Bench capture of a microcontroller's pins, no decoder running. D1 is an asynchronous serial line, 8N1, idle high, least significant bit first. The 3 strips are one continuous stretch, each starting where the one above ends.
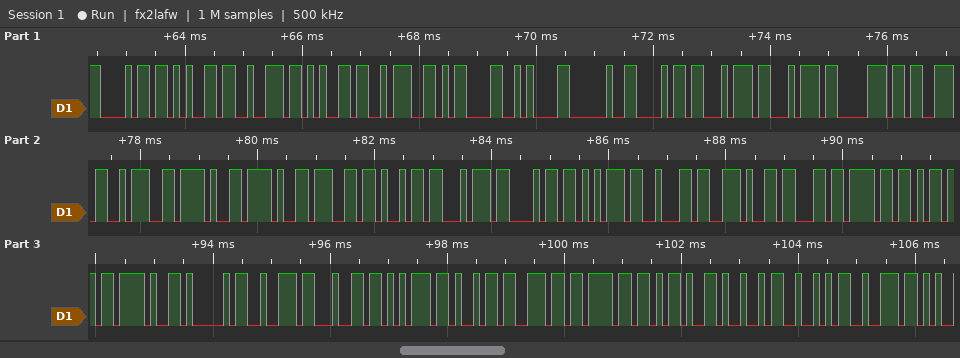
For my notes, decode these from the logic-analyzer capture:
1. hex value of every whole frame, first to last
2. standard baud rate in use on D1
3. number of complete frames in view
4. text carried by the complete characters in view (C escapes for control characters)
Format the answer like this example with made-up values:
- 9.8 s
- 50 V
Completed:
- 0x68 0x65 0x72 0x65 0x3A 0x0D 0x0A 0x20 0x68 0x74 0x74 0x70 0x73 0x3A 0x2F 0x2F 0x67 0x69 0x74 0x68 0x75 0x62 0x2E 0x63 0x6F 0x6D 0x2F 0x41 0x72 0x64 0x75 0x69 0x6E 0x6F 0x2D 0x49 0x52 0x72
- 9600 baud
- 38
- "here:\r\n https://github.com/Arduino-IRr"
